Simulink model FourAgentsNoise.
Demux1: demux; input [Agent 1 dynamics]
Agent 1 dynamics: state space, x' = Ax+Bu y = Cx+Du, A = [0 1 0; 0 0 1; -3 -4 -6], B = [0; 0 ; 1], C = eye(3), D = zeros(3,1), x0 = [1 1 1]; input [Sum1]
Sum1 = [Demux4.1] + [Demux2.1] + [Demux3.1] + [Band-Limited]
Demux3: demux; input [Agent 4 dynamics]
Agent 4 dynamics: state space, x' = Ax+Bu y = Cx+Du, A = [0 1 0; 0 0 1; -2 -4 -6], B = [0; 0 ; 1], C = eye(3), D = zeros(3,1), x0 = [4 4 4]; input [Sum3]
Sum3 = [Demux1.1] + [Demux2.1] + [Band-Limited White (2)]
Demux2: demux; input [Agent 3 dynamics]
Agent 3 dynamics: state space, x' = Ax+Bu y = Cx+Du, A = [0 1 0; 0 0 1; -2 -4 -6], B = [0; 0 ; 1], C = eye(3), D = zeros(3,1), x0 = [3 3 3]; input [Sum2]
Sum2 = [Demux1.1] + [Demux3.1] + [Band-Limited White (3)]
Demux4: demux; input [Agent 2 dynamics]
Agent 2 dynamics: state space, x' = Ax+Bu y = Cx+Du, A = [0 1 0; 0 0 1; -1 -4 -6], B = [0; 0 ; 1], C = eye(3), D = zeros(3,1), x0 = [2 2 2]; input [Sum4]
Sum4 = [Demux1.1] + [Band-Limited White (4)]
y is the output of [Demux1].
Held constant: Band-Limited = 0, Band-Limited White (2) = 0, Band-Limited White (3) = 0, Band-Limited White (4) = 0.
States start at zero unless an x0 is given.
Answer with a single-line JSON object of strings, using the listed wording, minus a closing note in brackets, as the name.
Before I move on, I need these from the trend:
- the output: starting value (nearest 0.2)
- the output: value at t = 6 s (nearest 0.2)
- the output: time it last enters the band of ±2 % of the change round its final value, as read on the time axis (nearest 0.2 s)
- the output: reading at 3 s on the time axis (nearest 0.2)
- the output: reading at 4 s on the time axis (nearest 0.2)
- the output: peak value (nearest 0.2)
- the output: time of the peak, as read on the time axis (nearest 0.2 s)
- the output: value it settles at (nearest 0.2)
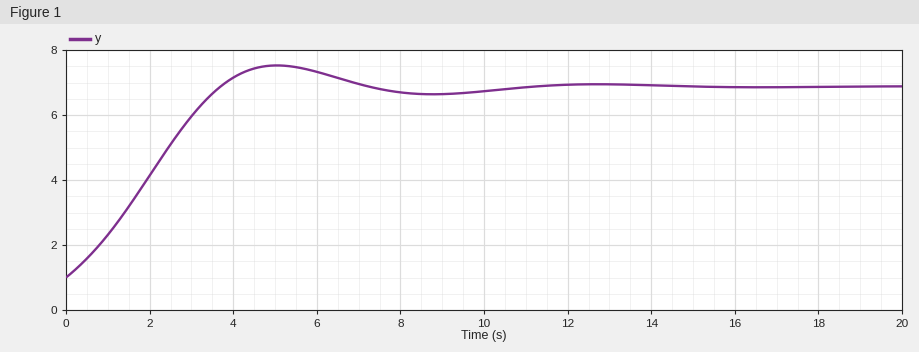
{"the output: starting value": "1.0", "the output: value at t = 6 s": "7.4", "the output: time it last enters the band of ±2 % of the change round its final value, as read on the time axis": "10.2 s", "the output: reading at 3 s on the time axis": "6.0", "the output: reading at 4 s on the time axis": "7.2", "the output: peak value": "7.6", "the output: time of the peak, as read on the time axis": "5.0 s", "the output: value it settles at": "6.8"}
